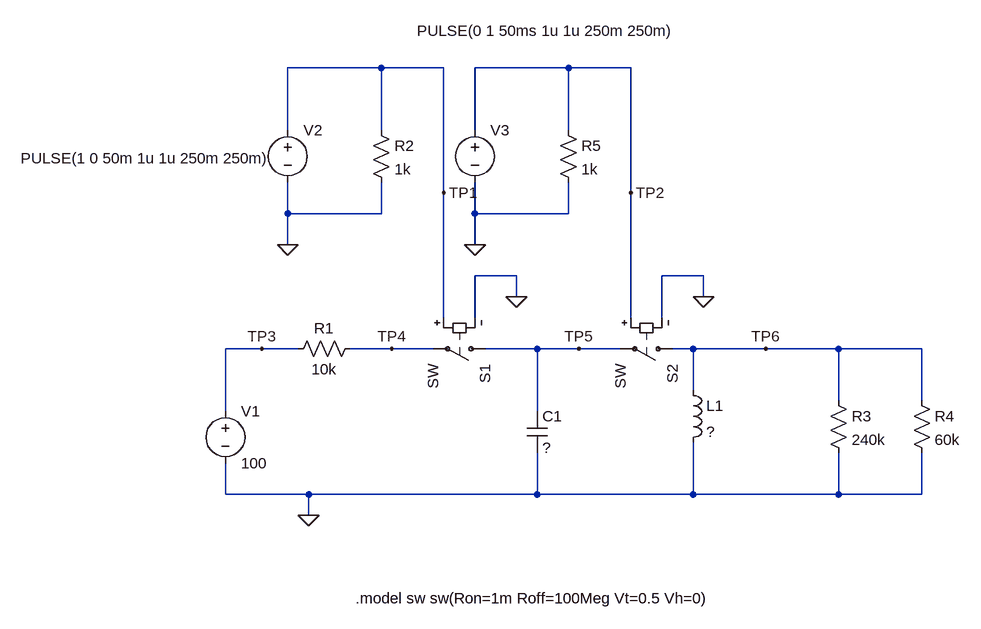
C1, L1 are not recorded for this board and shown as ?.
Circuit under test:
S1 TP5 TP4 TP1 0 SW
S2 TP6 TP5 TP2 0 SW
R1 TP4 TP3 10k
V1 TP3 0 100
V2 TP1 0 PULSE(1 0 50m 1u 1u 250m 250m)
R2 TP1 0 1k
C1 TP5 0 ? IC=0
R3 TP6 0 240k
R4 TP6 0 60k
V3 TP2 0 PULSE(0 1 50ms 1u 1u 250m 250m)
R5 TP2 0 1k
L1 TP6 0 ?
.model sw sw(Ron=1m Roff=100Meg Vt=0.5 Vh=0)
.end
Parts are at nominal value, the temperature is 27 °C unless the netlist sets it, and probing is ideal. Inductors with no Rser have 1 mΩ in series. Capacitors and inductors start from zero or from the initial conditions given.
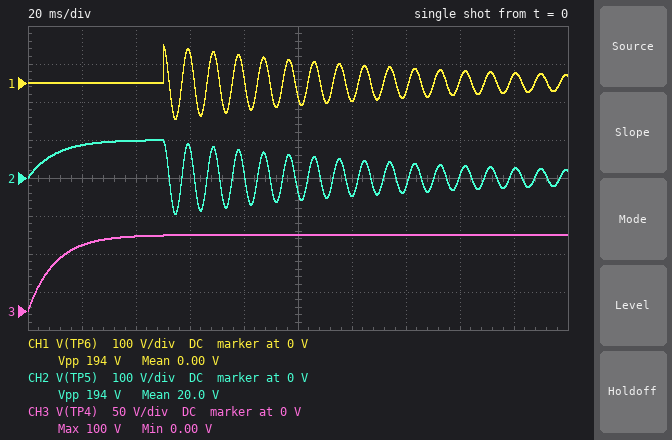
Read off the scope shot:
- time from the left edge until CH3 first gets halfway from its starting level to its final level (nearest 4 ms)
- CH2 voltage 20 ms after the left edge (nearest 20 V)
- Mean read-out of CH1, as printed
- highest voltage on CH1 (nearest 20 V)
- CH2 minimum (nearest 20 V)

8 ms
80 V
0.00 V
100 V
-100 V
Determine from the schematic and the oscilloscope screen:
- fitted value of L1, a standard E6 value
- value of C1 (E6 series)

2.2 H
1 µF
